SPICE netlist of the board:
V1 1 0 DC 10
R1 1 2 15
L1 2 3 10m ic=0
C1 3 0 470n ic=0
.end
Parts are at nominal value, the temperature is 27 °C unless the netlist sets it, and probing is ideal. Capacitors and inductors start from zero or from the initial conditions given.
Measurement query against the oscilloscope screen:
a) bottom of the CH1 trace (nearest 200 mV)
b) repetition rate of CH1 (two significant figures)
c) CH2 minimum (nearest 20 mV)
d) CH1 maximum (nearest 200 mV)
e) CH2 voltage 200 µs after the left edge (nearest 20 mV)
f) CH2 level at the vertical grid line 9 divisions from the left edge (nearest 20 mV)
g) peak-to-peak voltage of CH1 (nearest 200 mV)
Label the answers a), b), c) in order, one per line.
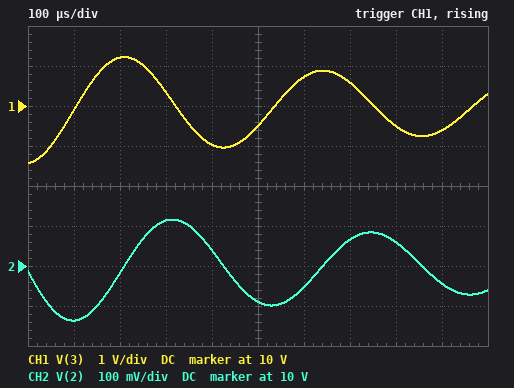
a) 8.6 V
b) 2.3 kHz
c) 9.86 V
d) 11.2 V
e) 9.98 V
f) 9.96 V
g) 2.6 V
